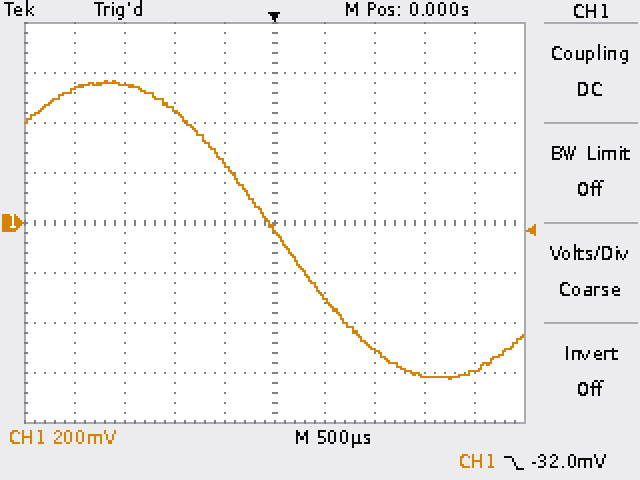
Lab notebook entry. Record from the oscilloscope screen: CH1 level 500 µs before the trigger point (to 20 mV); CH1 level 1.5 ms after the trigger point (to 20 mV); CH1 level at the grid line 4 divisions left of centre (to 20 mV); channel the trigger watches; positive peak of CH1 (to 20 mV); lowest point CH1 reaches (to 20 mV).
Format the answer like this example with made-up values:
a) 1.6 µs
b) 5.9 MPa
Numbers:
a) 240 mV
b) -620 mV
c) 540 mV
d) CH1
e) 560 mV
f) -620 mV
